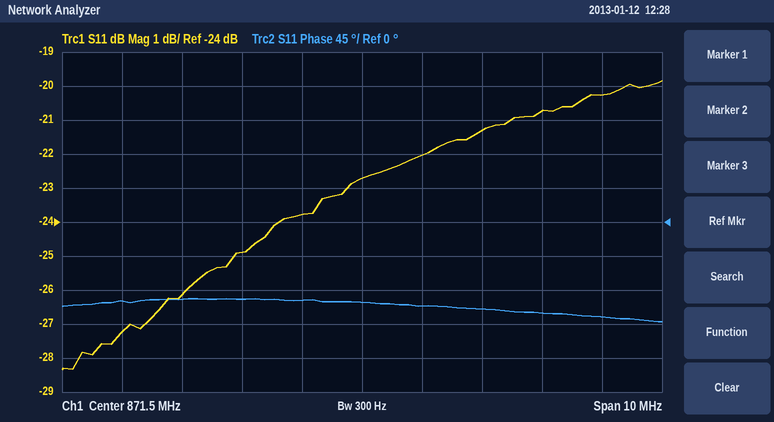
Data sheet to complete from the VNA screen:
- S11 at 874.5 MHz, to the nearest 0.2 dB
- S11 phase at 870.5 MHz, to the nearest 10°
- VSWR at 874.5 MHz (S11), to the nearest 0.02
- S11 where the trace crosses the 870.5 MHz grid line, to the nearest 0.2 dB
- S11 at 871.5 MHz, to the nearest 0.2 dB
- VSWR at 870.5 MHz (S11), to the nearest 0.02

-20.8 dB
-100°
1.20
-23.8 dB
-22.8 dB
1.14
